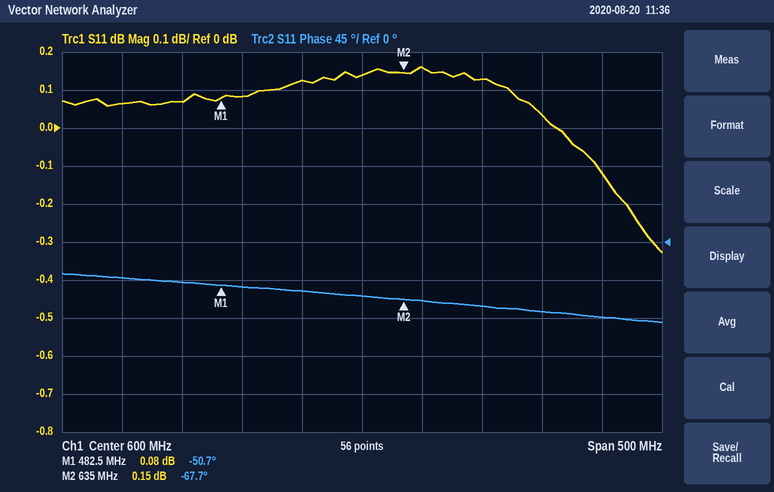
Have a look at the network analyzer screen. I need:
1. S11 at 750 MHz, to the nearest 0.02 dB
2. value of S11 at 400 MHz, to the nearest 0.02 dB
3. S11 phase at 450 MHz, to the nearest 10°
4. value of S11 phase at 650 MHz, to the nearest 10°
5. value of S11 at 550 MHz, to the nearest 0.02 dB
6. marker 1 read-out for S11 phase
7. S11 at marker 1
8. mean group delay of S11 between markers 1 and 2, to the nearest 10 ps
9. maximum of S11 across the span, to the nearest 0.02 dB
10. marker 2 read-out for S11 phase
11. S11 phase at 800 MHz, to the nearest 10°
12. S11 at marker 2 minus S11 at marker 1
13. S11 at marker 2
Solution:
0.04 dB
0.06 dB
-50°
-70°
0.12 dB
-50.7°
0.08 dB
310 ps
0.16 dB
-67.7°
-90°
0.07 dB
0.15 dB
